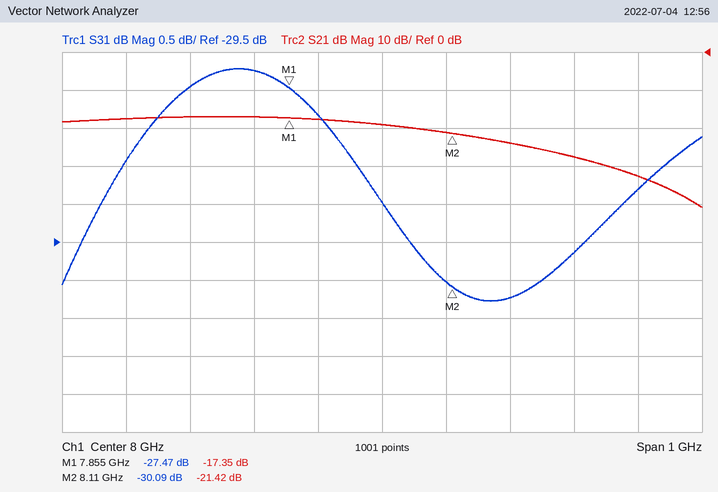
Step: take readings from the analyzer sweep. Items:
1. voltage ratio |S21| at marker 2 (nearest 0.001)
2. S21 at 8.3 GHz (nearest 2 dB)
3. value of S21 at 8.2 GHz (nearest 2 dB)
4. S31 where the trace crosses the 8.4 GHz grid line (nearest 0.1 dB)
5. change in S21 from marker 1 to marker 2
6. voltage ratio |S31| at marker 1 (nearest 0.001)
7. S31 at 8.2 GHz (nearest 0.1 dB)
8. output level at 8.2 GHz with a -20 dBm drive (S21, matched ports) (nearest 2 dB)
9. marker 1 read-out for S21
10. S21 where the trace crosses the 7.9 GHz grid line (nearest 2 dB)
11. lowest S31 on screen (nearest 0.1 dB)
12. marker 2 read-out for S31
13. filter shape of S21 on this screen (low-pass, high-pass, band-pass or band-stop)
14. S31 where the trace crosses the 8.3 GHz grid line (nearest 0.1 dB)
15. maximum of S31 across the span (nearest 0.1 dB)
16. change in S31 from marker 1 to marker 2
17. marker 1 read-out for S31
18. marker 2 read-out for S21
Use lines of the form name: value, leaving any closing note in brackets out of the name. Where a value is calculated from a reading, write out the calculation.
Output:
voltage ratio |S21| at marker 2: 10^(-21.42/20) ≈ 0.085
S21 at 8.3 GHz: -28 dB
value of S21 at 8.2 GHz: -24 dB
S31 where the trace crosses the 8.4 GHz grid line: -28.8 dB
change in S21 from marker 1 to marker 2: -21.42 − (-17.35) = -4.07 dB
voltage ratio |S31| at marker 1: 10^(-27.47/20) ≈ 0.042
S31 at 8.2 GHz: -30.2 dB
output level at 8.2 GHz with a -20 dBm drive (S21, matched ports): -20 dBm + (-24 dB) = -44 dBm
marker 1 read-out for S21: -17.35 dB
S21 where the trace crosses the 7.9 GHz grid line: -18 dB
lowest S31 on screen: -30.3 dB
marker 2 read-out for S31: -30.09 dB
filter shape of S21 on this screen: low-pass
S31 where the trace crosses the 8.3 GHz grid line: -29.6 dB
maximum of S31 across the span: -27.2 dB
change in S31 from marker 1 to marker 2: -30.09 − (-27.47) = -2.62 dB
marker 1 read-out for S31: -27.47 dB
marker 2 read-out for S21: -21.42 dB
